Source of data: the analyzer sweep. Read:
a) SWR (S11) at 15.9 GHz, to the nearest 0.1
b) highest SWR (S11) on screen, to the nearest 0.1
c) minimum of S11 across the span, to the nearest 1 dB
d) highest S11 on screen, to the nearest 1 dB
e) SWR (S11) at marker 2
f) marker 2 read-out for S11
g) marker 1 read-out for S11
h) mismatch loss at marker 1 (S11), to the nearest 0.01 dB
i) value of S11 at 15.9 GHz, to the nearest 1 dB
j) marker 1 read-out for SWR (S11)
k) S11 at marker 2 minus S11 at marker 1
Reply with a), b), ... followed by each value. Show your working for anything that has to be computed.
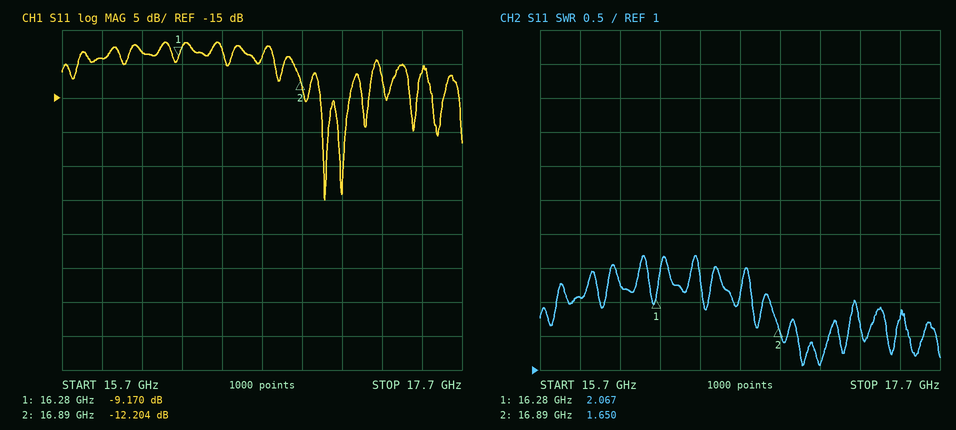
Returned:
a) 2.1
b) 2.7
c) -30 dB
d) -7 dB
e) 1.650
f) -12.204 dB
g) -9.170 dB
h) −10 log10(1 − 10^(-9.17/10)) ≈ 0.56 dB
i) -9 dB
j) 2.067
k) -12.204 − (-9.17) = -3.034 dB
